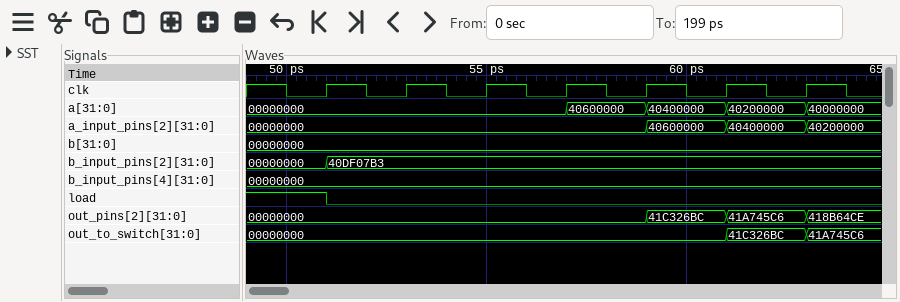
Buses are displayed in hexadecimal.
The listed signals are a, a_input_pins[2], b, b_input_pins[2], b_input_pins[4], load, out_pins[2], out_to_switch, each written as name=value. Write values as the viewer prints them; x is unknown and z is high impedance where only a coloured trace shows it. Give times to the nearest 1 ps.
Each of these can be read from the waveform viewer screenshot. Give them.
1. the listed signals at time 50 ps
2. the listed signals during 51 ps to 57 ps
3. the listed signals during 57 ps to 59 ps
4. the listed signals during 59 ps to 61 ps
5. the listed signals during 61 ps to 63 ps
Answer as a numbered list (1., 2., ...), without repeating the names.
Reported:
1. a=00000000, a_input_pins[2]=00000000, b=00000000, b_input_pins[2]=00000000, b_input_pins[4]=00000000, load=1, out_pins[2]=00000000, out_to_switch=00000000
2. a=00000000, a_input_pins[2]=00000000, b=00000000, b_input_pins[2]=40DF07B3, b_input_pins[4]=00000000, load=0, out_pins[2]=00000000, out_to_switch=00000000
3. a=40600000, a_input_pins[2]=00000000, b=00000000, b_input_pins[2]=40DF07B3, b_input_pins[4]=00000000, load=0, out_pins[2]=00000000, out_to_switch=00000000
4. a=40400000, a_input_pins[2]=40600000, b=00000000, b_input_pins[2]=40DF07B3, b_input_pins[4]=00000000, load=0, out_pins[2]=41C326BC, out_to_switch=00000000
5. a=40200000, a_input_pins[2]=40400000, b=00000000, b_input_pins[2]=40DF07B3, b_input_pins[4]=00000000, load=0, out_pins[2]=41A745C6, out_to_switch=41C326BC
